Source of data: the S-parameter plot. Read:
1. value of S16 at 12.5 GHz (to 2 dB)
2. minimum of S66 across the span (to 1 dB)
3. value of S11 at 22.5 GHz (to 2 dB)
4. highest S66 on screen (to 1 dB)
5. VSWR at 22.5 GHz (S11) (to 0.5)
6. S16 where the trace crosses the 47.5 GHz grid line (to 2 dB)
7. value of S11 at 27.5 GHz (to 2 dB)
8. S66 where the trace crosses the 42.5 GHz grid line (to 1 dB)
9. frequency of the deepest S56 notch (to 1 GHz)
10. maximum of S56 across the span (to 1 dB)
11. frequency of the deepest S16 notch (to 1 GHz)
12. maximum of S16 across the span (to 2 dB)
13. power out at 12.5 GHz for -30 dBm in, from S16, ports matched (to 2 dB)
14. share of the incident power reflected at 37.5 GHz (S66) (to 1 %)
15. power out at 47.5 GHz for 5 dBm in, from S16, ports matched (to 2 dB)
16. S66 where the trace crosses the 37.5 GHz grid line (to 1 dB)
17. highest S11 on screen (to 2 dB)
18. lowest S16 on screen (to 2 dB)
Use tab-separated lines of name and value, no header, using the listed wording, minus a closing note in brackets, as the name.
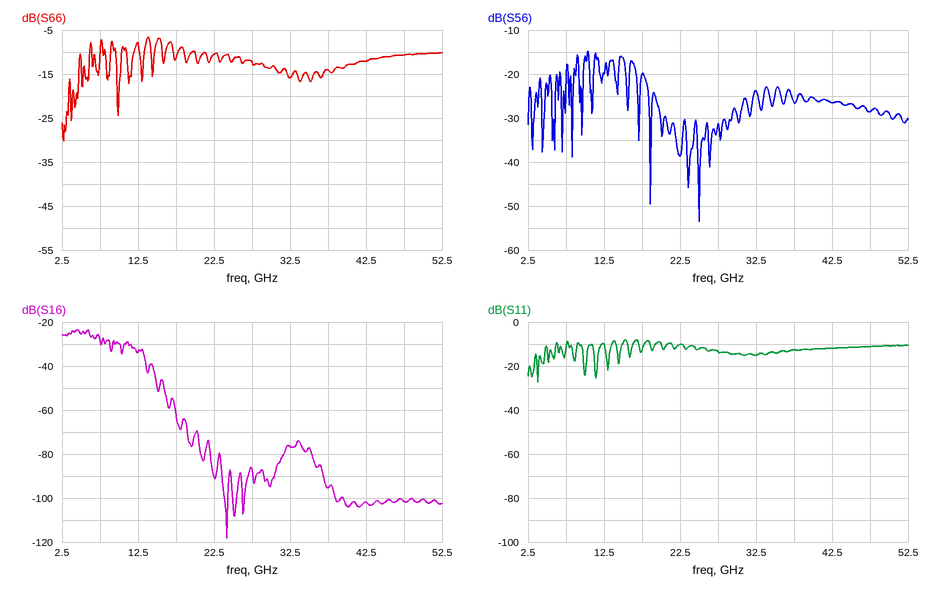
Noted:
value of S16 at 12.5 GHz	-34 dB
minimum of S66 across the span	-30 dB
value of S11 at 22.5 GHz	-10 dB
highest S66 on screen	-7 dB
VSWR at 22.5 GHz (S11)	2.0
S16 where the trace crosses the 47.5 GHz grid line	-102 dB
value of S11 at 27.5 GHz	-14 dB
S66 where the trace crosses the 42.5 GHz grid line	-12 dB
frequency of the deepest S56 notch	25 GHz
maximum of S56 across the span	-15 dB
frequency of the deepest S16 notch	24 GHz
maximum of S16 across the span	-24 dB
power out at 12.5 GHz for -30 dBm in, from S16, ports matched	-64 dBm
share of the incident power reflected at 37.5 GHz (S66)	4 %
power out at 47.5 GHz for 5 dBm in, from S16, ports matched	-96 dBm
S66 where the trace crosses the 37.5 GHz grid line	-14 dB
highest S11 on screen	-8 dB
lowest S16 on screen	-118 dB
